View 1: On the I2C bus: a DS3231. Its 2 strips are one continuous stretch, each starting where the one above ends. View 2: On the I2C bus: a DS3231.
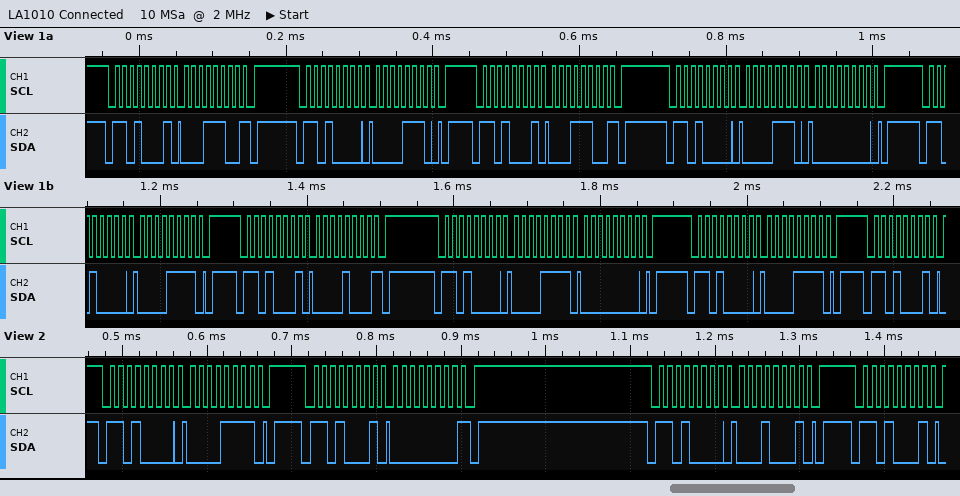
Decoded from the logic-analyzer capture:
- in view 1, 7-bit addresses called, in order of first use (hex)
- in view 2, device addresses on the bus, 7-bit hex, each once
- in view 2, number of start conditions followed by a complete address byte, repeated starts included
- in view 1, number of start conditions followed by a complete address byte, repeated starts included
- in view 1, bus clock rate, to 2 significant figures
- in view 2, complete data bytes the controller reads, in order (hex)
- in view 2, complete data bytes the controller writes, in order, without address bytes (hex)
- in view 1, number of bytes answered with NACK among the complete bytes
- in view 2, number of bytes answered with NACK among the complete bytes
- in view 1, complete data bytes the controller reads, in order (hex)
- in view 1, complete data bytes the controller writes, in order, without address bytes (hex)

0x68
0x68
4
9
100 kHz
00
0F 11
3
1
1C 1C 08
0E 0E 00 0F 0F 00 0F
